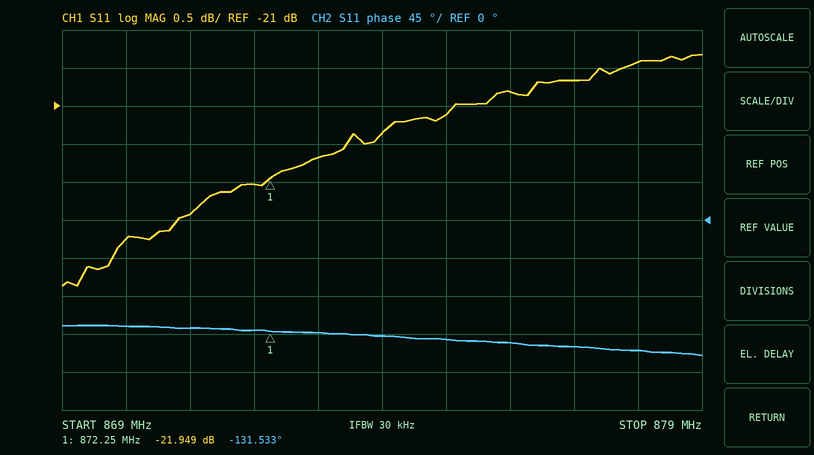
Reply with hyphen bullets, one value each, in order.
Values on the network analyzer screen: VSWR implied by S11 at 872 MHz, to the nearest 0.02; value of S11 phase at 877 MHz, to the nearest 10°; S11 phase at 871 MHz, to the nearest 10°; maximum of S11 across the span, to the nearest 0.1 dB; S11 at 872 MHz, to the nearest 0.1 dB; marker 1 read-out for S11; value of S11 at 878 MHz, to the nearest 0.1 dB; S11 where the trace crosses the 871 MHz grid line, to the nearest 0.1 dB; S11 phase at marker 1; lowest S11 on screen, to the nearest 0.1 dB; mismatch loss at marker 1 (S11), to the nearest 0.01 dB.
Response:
- 1.18
- -150°
- -130°
- -20.3 dB
- -22.0 dB
- -21.949 dB
- -20.4 dB
- -22.4 dB
- -131.533°
- -23.4 dB
- 0.03 dB
